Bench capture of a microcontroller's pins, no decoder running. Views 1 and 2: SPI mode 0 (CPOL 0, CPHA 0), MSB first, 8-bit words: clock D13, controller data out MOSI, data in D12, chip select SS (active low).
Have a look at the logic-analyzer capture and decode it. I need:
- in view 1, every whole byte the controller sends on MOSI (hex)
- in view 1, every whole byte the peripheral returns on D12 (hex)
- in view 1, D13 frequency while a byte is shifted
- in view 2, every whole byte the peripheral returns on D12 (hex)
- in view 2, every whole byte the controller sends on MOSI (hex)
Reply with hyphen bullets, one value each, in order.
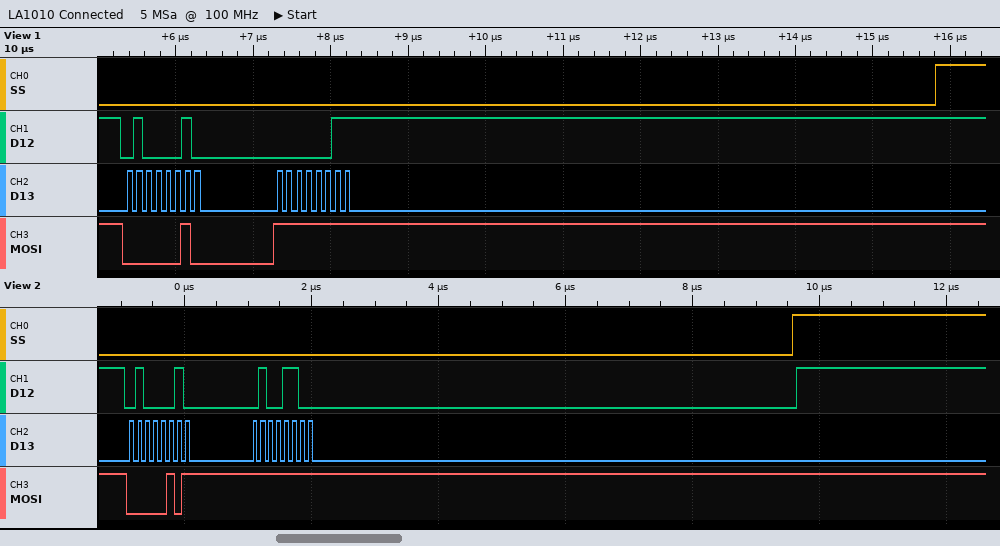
- 0x02 0xFF
- 0x42 0x03
- 8 MHz
- 42 4C
- 05 FF
